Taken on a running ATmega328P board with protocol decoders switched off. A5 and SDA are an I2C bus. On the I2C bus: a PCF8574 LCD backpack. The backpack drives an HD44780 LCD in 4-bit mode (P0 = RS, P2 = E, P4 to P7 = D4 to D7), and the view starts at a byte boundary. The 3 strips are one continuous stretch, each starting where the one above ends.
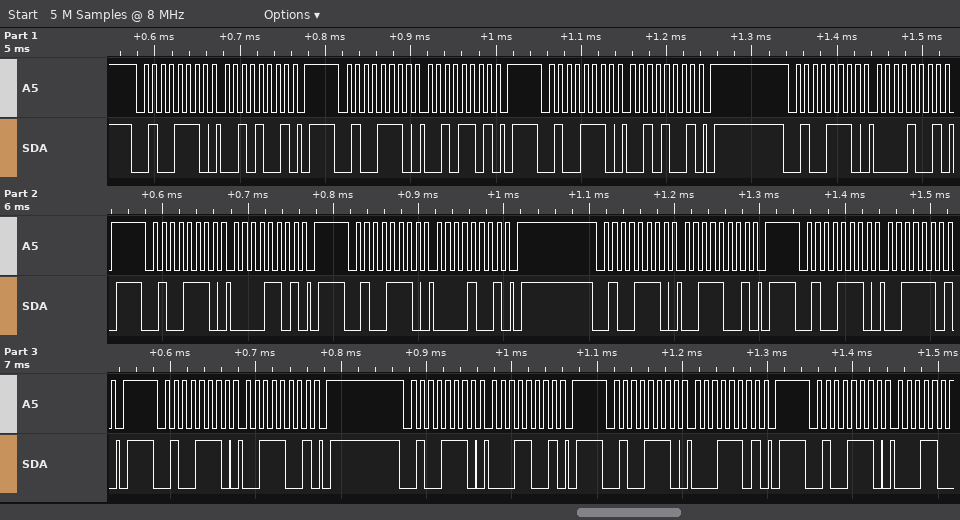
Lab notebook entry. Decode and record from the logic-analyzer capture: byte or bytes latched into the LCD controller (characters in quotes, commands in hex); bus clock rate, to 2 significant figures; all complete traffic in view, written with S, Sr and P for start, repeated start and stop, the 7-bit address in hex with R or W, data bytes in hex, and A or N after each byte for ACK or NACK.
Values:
' '
100 kHz
S 27W A 29 A P S 27W A 2D A P S 27W A 29 A P S 27W A 09 A P S 27W A 0D A P S 27W A 09 A P S 27W A 39 A P S 27W A 3D A P S 27W A 39 A P S 27W A 19 A P S 27W A 1D A P S 27W A
